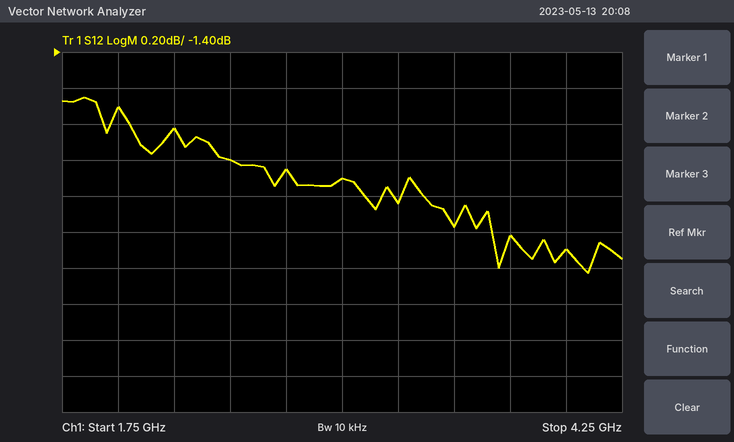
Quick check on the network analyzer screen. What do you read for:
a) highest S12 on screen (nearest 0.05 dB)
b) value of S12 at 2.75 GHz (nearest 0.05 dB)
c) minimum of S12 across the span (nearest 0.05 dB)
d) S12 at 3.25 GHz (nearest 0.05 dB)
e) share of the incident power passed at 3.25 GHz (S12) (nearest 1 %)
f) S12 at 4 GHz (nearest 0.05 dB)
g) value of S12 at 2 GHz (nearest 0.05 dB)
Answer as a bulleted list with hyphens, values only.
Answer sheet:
- -1.65 dB
- -2.05 dB
- -2.65 dB
- -2.25 dB
- 60 %
- -2.50 dB
- -1.70 dB
